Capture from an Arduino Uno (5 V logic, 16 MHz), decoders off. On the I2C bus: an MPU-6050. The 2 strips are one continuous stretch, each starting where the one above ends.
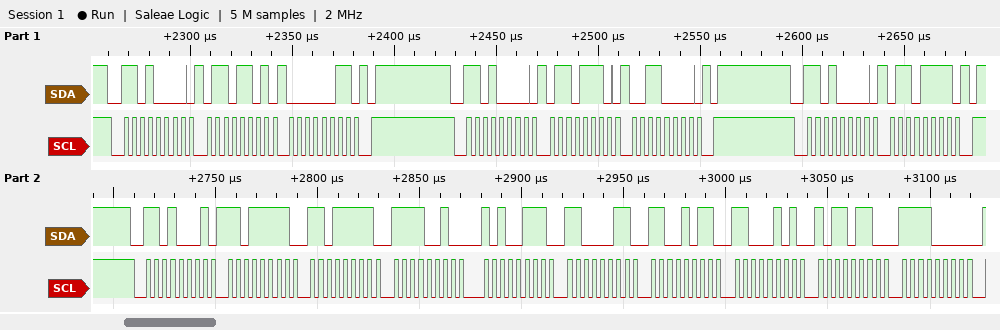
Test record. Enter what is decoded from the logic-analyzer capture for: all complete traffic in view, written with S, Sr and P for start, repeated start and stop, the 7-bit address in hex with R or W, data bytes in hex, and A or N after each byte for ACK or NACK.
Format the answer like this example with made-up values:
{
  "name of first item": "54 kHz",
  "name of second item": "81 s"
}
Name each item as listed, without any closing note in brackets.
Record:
{
  "all complete traffic in view, written with S, Sr and P for start, repeated start and stop, the 7-bit address in hex with R or W, data bytes in hex, and A or N after each byte for ACK or NACK": "S 68W A 6D A 03 A P S 68W A 6E A 30 A P S 68W A 6F A P S 68R A DF A DF A F2 A A7 A C3 A CB A C5 A B6 A F0 A"
}
